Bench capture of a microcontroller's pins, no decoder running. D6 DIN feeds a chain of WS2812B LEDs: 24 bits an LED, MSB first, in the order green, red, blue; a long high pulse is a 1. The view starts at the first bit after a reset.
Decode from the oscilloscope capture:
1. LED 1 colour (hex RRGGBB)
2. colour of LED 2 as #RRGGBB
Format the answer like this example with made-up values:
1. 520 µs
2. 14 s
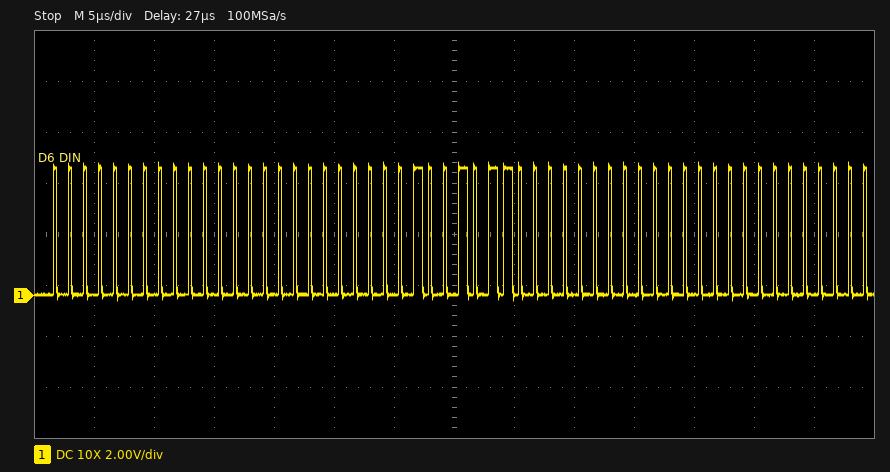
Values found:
1. #000000
2. #009600
